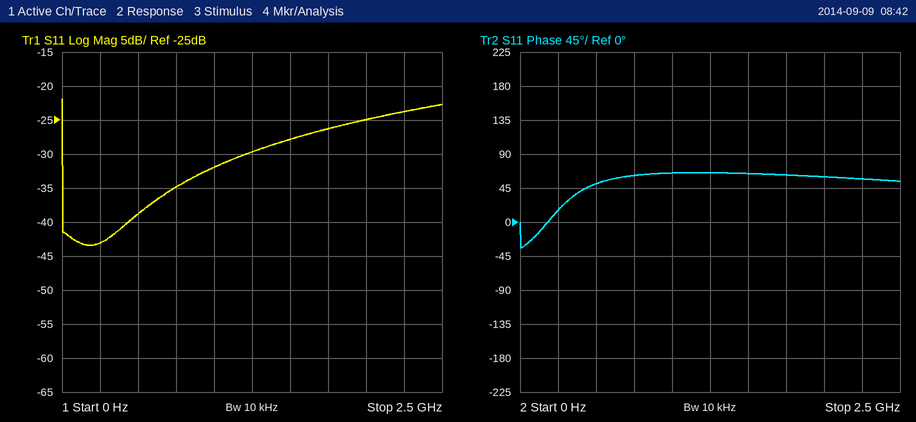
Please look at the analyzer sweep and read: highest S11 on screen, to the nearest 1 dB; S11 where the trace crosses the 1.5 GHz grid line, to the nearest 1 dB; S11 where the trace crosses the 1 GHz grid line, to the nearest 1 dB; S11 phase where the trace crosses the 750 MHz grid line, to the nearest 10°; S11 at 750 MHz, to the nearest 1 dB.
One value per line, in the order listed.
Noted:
-22 dB
-28 dB
-32 dB
60°
-35 dB
